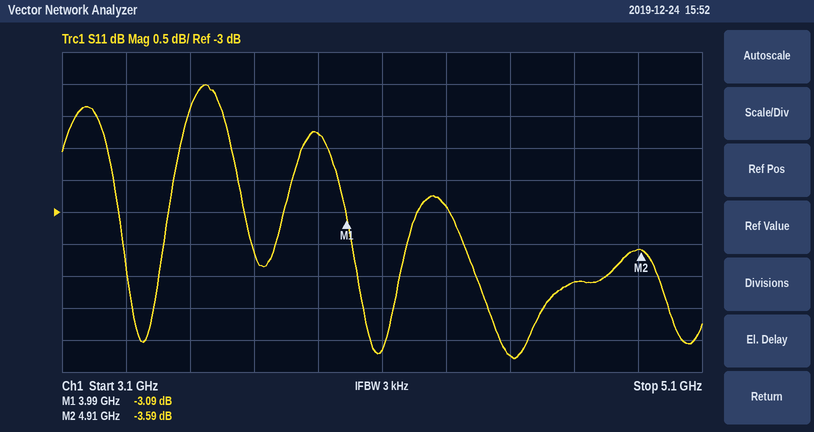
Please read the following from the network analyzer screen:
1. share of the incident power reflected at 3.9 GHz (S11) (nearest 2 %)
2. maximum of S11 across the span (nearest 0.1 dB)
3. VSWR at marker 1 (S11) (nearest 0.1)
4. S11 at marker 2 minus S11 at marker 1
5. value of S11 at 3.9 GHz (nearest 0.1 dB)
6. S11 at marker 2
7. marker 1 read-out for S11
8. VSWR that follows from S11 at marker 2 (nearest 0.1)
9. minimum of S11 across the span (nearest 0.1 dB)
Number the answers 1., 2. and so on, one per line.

1. 66 %
2. -1.0 dB
3. 5.7
4. -0.50 dB
5. -1.8 dB
6. -3.59 dB
7. -3.09 dB
8. 4.9
9. -5.3 dB
